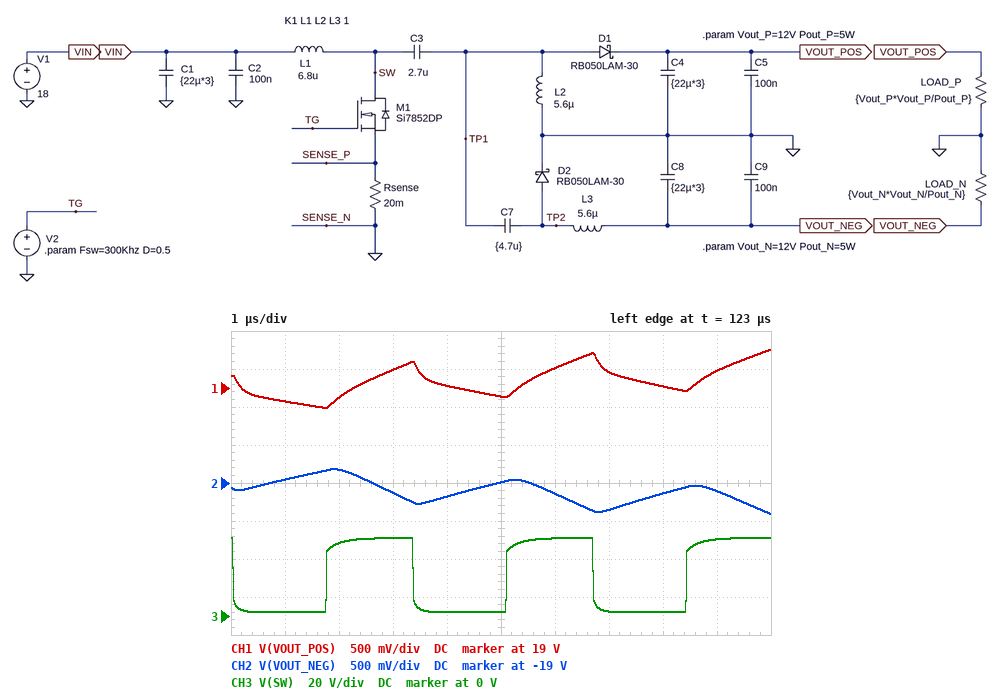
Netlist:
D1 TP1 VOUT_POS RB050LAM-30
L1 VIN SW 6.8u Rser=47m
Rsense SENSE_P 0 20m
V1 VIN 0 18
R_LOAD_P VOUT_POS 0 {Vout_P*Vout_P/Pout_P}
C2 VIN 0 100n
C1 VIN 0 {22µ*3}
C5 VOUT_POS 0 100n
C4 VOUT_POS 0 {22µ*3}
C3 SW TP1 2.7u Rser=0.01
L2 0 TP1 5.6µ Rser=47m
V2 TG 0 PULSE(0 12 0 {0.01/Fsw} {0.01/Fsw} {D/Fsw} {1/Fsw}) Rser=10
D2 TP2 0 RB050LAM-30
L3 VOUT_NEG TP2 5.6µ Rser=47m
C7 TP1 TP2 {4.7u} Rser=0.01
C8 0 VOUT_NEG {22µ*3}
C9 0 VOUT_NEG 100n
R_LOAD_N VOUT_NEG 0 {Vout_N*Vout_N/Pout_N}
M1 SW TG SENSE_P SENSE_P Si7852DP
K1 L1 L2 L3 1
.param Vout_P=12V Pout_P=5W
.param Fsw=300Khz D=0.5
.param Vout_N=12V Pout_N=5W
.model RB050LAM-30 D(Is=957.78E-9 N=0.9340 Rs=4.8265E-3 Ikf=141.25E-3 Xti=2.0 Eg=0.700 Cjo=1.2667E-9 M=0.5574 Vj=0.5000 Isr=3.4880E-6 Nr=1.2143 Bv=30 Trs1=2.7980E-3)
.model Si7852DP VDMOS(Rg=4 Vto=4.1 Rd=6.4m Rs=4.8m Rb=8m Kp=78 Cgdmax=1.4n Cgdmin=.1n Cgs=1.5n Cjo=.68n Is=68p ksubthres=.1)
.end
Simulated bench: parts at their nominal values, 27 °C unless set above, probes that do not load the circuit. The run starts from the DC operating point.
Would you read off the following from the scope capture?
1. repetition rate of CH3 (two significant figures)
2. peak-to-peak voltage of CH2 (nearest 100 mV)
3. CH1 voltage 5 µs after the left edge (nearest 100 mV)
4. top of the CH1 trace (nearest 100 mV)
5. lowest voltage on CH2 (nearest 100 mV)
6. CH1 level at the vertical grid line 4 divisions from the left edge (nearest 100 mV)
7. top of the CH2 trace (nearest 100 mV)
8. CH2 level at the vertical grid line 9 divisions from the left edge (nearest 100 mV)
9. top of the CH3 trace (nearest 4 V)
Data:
300 kHz
600 mV
18.9 V
19.5 V
-19.4 V
19.0 V
-18.8 V
-19.1 V
40 V
